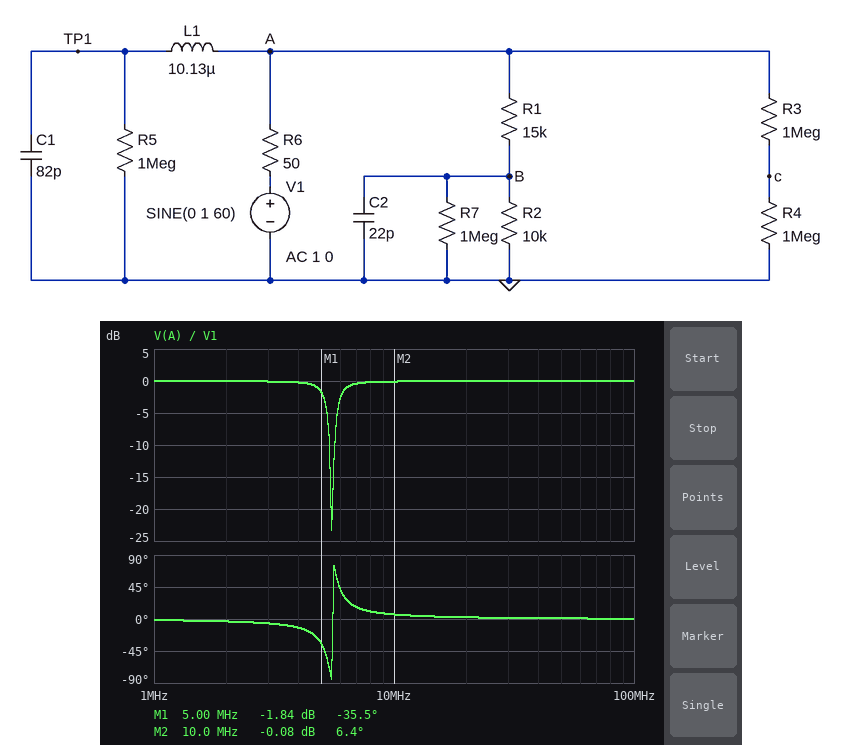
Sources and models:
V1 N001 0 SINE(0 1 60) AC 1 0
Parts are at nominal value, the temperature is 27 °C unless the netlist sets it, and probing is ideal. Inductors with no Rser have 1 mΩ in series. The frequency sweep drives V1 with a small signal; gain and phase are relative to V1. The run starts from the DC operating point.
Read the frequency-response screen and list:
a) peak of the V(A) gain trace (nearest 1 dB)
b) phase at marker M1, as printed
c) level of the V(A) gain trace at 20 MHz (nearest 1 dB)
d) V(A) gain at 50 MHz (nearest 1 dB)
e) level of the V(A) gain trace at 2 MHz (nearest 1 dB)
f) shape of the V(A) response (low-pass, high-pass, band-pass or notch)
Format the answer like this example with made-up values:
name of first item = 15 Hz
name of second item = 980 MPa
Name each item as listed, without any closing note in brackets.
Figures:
peak of the V(A) gain trace = 0 dB
phase at marker M1, as printed = -35.5 deg
level of the V(A) gain trace at 20 MHz = 0 dB
V(A) gain at 50 MHz = 0 dB
level of the V(A) gain trace at 2 MHz = 0 dB
shape of the V(A) response = notch
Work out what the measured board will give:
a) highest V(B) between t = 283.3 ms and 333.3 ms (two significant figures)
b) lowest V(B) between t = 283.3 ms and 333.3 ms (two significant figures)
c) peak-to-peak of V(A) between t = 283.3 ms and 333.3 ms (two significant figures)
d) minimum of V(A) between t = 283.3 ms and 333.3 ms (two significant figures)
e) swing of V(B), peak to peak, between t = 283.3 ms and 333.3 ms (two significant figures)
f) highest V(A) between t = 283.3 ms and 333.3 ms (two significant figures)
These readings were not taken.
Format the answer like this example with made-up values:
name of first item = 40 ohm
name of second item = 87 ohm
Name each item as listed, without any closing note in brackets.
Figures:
highest V(B) between t = 283.3 ms and 333.3 ms = 400 mV
lowest V(B) between t = 283.3 ms and 333.3 ms = -400 mV
peak-to-peak of V(A) between t = 283.3 ms and 333.3 ms = 2.0 V
minimum of V(A) between t = 283.3 ms and 333.3 ms = -1.0 V
swing of V(B), peak to peak, between t = 283.3 ms and 333.3 ms = 790 mV
highest V(A) between t = 283.3 ms and 333.3 ms = 1.0 V
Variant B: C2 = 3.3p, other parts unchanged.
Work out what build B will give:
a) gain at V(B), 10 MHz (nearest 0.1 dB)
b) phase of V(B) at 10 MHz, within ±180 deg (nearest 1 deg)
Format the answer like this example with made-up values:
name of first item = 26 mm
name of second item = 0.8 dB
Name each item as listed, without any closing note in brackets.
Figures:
gain at V(B), 10 MHz = -12.1 dB
phase of V(B) at 10 MHz, within ±180 deg = -45 deg
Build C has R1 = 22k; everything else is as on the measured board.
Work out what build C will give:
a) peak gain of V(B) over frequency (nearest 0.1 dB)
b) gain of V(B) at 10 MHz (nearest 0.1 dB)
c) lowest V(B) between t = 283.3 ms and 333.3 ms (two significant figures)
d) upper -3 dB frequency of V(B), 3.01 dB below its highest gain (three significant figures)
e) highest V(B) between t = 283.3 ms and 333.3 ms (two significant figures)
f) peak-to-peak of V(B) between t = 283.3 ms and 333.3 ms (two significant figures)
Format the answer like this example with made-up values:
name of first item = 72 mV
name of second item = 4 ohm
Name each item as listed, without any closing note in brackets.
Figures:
peak gain of V(B) over frequency = -10.2 dB
gain of V(B) at 10 MHz = -29.8 dB
lowest V(B) between t = 283.3 ms and 333.3 ms = -310 mV
upper -3 dB frequency of V(B), 3.01 dB below its highest gain = 1.06 MHz
highest V(B) between t = 283.3 ms and 333.3 ms = 310 mV
peak-to-peak of V(B) between t = 283.3 ms and 333.3 ms = 620 mV
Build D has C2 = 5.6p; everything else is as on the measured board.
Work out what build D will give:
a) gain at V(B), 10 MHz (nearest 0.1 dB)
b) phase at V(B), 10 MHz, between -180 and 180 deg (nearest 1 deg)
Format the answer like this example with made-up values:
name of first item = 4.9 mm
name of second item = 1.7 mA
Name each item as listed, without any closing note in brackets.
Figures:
gain at V(B), 10 MHz = -15.4 dB
phase at V(B), 10 MHz, between -180 and 180 deg = -58 deg
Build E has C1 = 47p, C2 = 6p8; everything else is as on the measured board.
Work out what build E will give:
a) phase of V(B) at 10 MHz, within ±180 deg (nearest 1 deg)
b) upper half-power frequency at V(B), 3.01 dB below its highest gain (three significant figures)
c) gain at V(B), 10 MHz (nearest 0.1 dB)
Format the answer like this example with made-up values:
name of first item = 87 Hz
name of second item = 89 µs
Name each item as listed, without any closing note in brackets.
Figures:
phase of V(B) at 10 MHz, within ±180 deg = -59 deg
upper half-power frequency at V(B), 3.01 dB below its highest gain = 3.89 MHz
gain at V(B), 10 MHz = -16.9 dB
